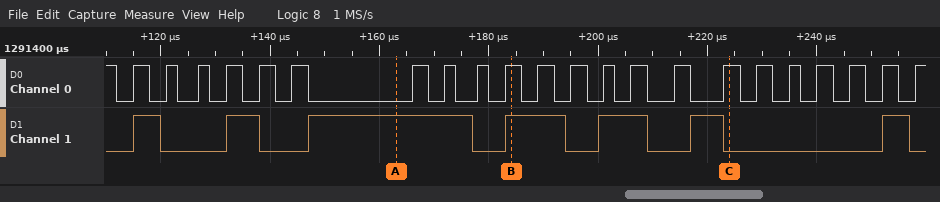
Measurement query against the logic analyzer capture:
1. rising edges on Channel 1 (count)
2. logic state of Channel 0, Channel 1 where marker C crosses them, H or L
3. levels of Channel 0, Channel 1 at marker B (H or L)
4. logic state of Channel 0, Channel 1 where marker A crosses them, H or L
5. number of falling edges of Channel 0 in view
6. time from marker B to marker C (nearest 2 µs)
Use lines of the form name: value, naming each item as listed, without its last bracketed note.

rising edges on Channel 1: 7
logic state of Channel 0, Channel 1 where marker C crosses them, H or L: Channel 0=H, Channel 1=L
levels of Channel 0, Channel 1 at marker B: Channel 0=H, Channel 1=H
logic state of Channel 0, Channel 1 where marker A crosses them, H or L: Channel 0=L, Channel 1=H
number of falling edges of Channel 0 in view: 22
time from marker B to marker C: 40 µs
